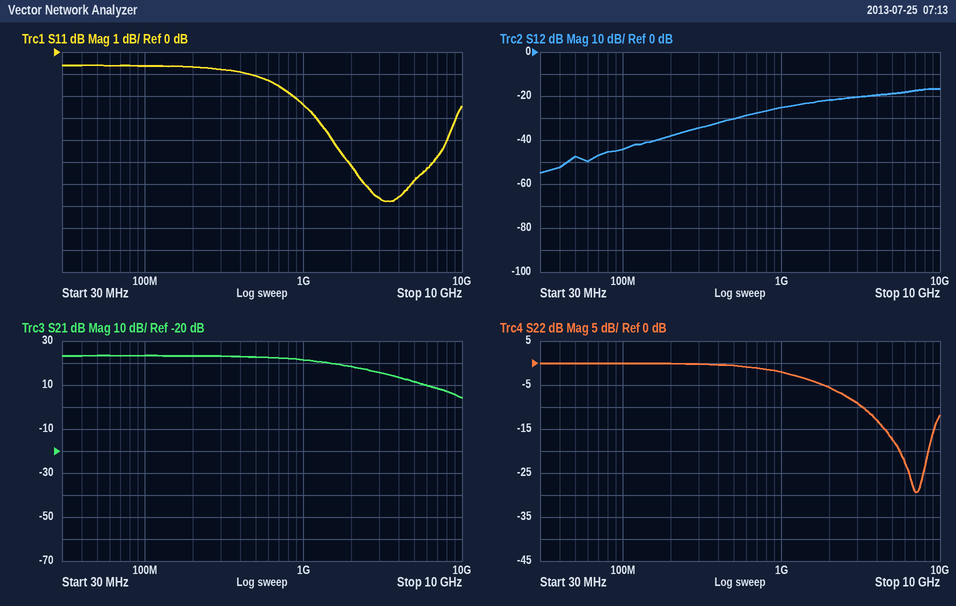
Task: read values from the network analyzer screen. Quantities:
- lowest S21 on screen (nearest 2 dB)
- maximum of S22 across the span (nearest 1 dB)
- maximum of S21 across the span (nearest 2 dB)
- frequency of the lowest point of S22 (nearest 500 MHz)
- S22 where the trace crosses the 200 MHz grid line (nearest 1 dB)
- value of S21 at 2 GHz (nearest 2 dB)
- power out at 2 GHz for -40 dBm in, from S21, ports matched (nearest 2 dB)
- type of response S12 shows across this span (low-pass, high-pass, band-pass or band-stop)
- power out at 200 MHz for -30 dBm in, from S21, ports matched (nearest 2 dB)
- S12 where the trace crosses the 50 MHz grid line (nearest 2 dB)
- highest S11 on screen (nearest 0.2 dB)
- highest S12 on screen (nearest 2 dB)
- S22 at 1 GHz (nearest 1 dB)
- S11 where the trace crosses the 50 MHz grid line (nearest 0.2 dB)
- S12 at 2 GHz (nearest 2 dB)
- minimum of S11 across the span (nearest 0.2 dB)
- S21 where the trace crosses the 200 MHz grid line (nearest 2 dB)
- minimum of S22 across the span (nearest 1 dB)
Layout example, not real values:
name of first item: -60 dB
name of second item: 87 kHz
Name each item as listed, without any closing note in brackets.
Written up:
lowest S21 on screen: 4 dB
maximum of S22 across the span: 0 dB
maximum of S21 across the span: 24 dB
frequency of the lowest point of S22: 7.0 GHz
S22 where the trace crosses the 200 MHz grid line: 0 dB
value of S21 at 2 GHz: 18 dB
power out at 2 GHz for -40 dBm in, from S21, ports matched: -22 dBm
type of response S12 shows across this span: high-pass
power out at 200 MHz for -30 dBm in, from S21, ports matched: -6 dBm
S12 where the trace crosses the 50 MHz grid line: -48 dB
highest S11 on screen: -0.6 dB
highest S12 on screen: -16 dB
S22 at 1 GHz: -2 dB
S11 where the trace crosses the 50 MHz grid line: -0.6 dB
S12 at 2 GHz: -22 dB
minimum of S11 across the span: -6.8 dB
S21 where the trace crosses the 200 MHz grid line: 24 dB
minimum of S22 across the span: -29 dB
